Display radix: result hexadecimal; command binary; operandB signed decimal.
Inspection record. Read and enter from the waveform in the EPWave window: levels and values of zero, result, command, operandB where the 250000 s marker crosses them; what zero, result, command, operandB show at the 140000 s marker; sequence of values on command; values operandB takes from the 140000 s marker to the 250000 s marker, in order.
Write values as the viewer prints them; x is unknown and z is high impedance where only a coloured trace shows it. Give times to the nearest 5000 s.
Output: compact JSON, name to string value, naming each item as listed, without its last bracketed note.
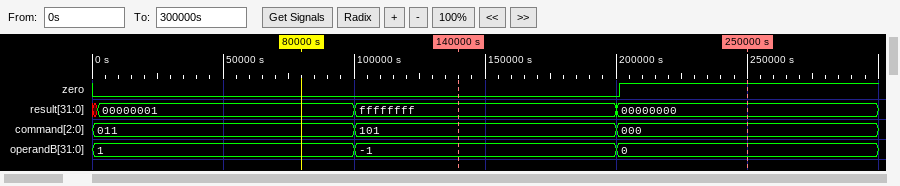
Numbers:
{"levels and values of zero, result, command, operandB where the 250000 s marker crosses them": "zero=1, result=00000000, command=000, operandB=0", "what zero, result, command, operandB show at the 140000 s marker": "zero=0, result=ffffffff, command=101, operandB=-1", "sequence of values on command": "011, 101, 000", "values operandB takes from the 140000 s marker to the 250000 s marker, in order": "-1, 0"}
